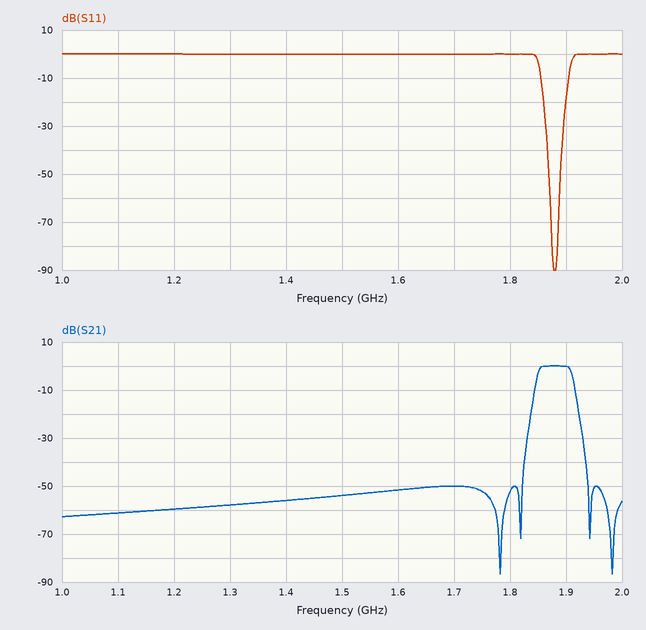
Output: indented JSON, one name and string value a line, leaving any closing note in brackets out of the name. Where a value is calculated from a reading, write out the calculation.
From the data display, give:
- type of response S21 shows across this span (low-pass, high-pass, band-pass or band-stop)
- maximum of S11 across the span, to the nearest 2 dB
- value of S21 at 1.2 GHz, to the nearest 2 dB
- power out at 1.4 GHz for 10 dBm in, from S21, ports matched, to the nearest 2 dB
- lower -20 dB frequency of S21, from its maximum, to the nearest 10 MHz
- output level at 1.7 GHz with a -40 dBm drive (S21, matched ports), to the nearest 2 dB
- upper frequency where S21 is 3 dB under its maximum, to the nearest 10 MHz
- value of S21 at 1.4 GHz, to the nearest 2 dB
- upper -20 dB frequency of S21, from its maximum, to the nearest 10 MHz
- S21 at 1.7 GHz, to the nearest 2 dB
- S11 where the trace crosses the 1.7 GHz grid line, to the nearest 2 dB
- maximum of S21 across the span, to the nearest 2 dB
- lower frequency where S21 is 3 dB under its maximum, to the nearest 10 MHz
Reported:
{
  "type of response S21 shows across this span": "band-pass",
  "maximum of S11 across the span, to the nearest 2 dB": "0 dB",
  "value of S21 at 1.2 GHz, to the nearest 2 dB": "-60 dB",
  "power out at 1.4 GHz for 10 dBm in, from S21, ports matched, to the nearest 2 dB": "10 dBm + (-56 dB) = -46 dBm",
  "lower -20 dB frequency of S21, from its maximum, to the nearest 10 MHz": "1.84 GHz",
  "output level at 1.7 GHz with a -40 dBm drive (S21, matched ports), to the nearest 2 dB": "-40 dBm + (-50 dB) = -90 dBm",
  "upper frequency where S21 is 3 dB under its maximum, to the nearest 10 MHz": "1.91 GHz",
  "value of S21 at 1.4 GHz, to the nearest 2 dB": "-56 dB",
  "upper -20 dB frequency of S21, from its maximum, to the nearest 10 MHz": "1.92 GHz",
  "S21 at 1.7 GHz, to the nearest 2 dB": "-50 dB",
  "S11 where the trace crosses the 1.7 GHz grid line, to the nearest 2 dB": "0 dB",
  "maximum of S21 across the span, to the nearest 2 dB": "0 dB",
  "lower frequency where S21 is 3 dB under its maximum, to the nearest 10 MHz": "1.85 GHz"
}
